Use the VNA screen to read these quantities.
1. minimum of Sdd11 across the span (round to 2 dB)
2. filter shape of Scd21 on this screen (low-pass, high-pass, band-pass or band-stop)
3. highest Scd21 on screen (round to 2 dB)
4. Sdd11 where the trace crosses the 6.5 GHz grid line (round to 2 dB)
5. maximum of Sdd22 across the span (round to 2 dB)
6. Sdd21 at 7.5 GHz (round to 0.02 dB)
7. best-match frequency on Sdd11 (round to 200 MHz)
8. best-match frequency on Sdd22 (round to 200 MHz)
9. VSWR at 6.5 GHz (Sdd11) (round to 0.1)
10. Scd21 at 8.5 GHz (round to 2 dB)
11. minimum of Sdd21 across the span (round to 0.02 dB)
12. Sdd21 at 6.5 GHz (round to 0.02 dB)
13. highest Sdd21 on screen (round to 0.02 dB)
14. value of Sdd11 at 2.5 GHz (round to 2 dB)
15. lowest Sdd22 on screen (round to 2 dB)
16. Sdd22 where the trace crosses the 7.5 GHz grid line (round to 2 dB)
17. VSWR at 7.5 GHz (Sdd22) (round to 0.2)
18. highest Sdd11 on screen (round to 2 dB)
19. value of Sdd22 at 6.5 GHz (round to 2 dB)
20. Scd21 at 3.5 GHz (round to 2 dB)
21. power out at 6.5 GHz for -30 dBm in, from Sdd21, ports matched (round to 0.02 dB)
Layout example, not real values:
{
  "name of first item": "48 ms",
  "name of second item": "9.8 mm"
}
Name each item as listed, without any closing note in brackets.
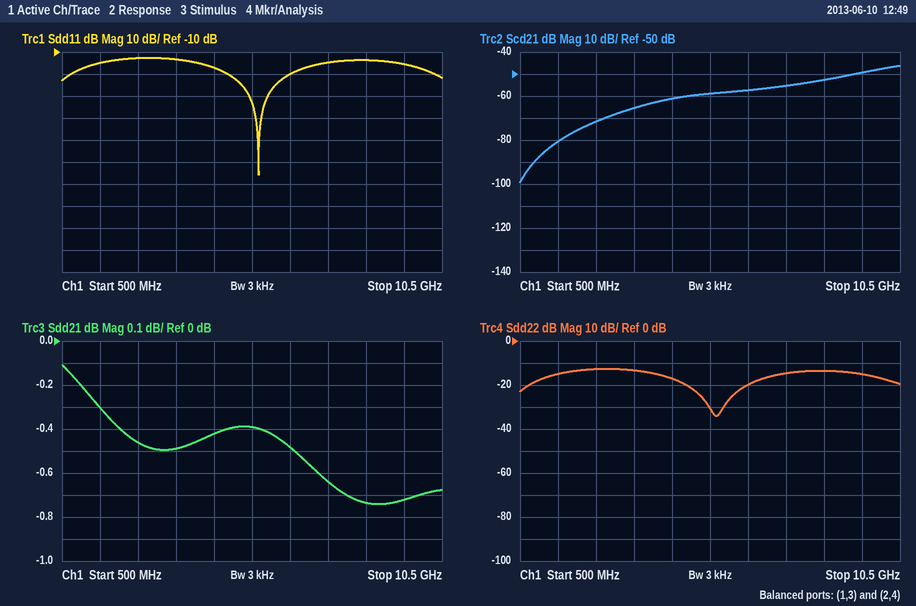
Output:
{
  "minimum of Sdd11 across the span": "-66 dB",
  "filter shape of Scd21 on this screen": "high-pass",
  "highest Scd21 on screen": "-46 dB",
  "Sdd11 where the trace crosses the 6.5 GHz grid line": "-20 dB",
  "maximum of Sdd22 across the span": "-12 dB",
  "Sdd21 at 7.5 GHz": "-0.64 dB",
  "best-match frequency on Sdd11": "5.6 GHz",
  "best-match frequency on Sdd22": "5.6 GHz",
  "VSWR at 6.5 GHz (Sdd11)": "1.2",
  "Scd21 at 8.5 GHz": "-52 dB",
  "minimum of Sdd21 across the span": "-0.74 dB",
  "Sdd21 at 6.5 GHz": "-0.48 dB",
  "highest Sdd21 on screen": "-0.10 dB",
  "value of Sdd11 at 2.5 GHz": "-12 dB",
  "lowest Sdd22 on screen": "-34 dB",
  "Sdd22 where the trace crosses the 7.5 GHz grid line": "-14 dB",
  "VSWR at 7.5 GHz (Sdd22)": "1.4",
  "highest Sdd11 on screen": "-12 dB",
  "value of Sdd22 at 6.5 GHz": "-20 dB",
  "Scd21 at 3.5 GHz": "-66 dB",
  "power out at 6.5 GHz for -30 dBm in, from Sdd21, ports matched": "-30.48 dBm"
}
